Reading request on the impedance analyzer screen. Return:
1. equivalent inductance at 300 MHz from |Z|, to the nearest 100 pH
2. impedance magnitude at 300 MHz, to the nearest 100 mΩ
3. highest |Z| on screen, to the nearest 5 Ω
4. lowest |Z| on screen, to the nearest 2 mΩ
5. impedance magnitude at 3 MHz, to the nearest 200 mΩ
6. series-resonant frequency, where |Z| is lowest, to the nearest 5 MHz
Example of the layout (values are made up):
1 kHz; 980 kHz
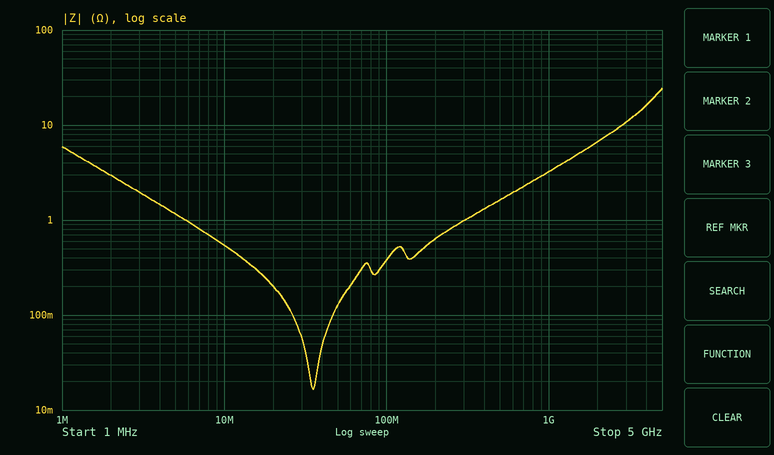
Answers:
500 pH; 1.0 Ω; 25 Ω; 16 mΩ; 2.0 Ω; 35 MHz
